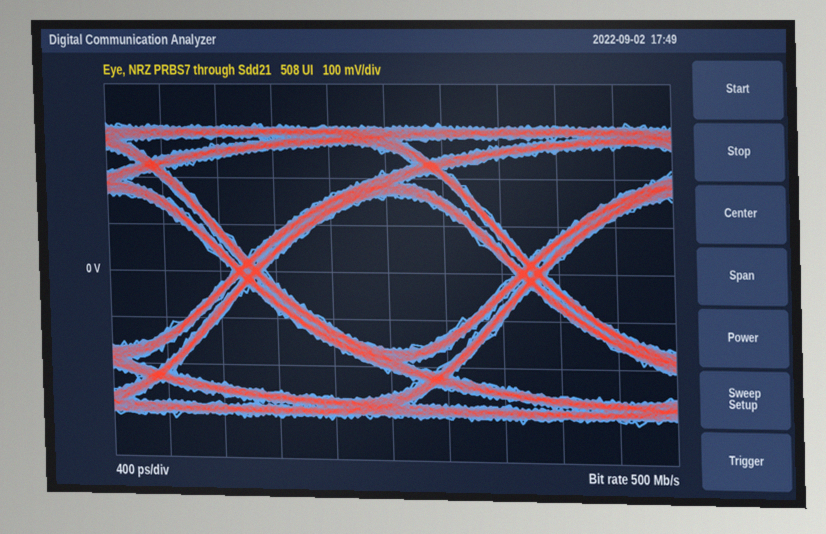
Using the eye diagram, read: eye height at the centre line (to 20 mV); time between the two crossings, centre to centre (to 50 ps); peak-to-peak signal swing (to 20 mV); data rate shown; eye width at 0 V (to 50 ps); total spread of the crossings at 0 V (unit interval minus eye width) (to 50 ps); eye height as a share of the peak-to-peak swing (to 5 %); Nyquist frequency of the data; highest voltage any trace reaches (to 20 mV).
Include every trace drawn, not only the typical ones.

320 mV
2.00 ns
640 mV
500 Mb/s
1.75 ns
250 ps
50 %
250 MHz
320 mV
